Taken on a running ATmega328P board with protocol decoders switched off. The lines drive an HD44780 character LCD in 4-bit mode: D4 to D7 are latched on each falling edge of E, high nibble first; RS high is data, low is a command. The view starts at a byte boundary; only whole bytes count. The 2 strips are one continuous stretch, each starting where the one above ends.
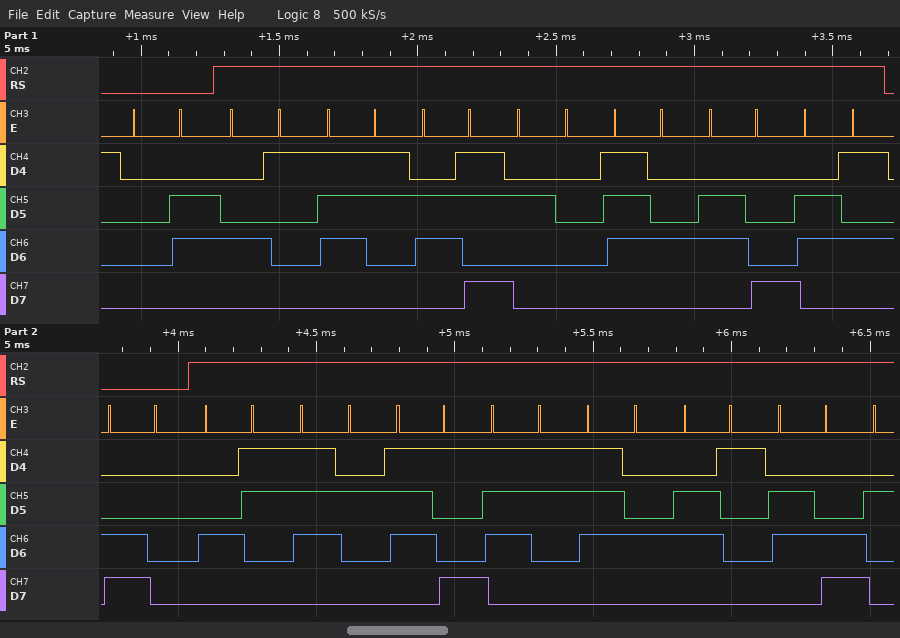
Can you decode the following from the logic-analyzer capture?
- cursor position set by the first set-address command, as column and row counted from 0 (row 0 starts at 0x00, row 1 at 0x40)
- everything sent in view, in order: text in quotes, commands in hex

column 0, row 1
0x06 "Ask the" 0xC0 "Crystal"
